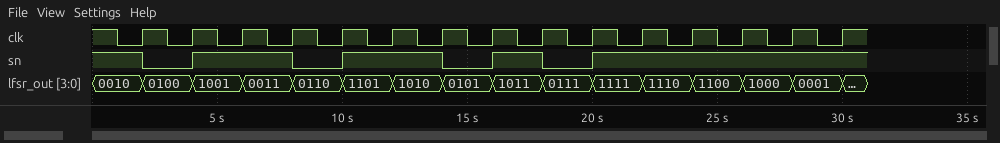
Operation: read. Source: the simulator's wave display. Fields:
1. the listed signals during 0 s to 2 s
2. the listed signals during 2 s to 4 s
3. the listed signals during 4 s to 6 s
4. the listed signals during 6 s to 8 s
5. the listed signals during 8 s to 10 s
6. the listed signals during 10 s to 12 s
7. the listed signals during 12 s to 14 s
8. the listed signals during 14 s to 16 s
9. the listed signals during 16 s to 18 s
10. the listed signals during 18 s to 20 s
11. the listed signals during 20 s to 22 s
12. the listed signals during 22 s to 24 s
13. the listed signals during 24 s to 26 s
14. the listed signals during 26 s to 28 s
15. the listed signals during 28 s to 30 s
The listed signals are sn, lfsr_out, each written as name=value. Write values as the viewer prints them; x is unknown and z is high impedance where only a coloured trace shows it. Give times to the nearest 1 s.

sn=1, lfsr_out=0010
sn=0, lfsr_out=0100
sn=1, lfsr_out=1001
sn=1, lfsr_out=0011
sn=0, lfsr_out=0110
sn=1, lfsr_out=1101
sn=1, lfsr_out=1010
sn=0, lfsr_out=0101
sn=1, lfsr_out=1011
sn=0, lfsr_out=0111
sn=1, lfsr_out=1111
sn=1, lfsr_out=1110
sn=1, lfsr_out=1100
sn=1, lfsr_out=1000
sn=1, lfsr_out=0001
